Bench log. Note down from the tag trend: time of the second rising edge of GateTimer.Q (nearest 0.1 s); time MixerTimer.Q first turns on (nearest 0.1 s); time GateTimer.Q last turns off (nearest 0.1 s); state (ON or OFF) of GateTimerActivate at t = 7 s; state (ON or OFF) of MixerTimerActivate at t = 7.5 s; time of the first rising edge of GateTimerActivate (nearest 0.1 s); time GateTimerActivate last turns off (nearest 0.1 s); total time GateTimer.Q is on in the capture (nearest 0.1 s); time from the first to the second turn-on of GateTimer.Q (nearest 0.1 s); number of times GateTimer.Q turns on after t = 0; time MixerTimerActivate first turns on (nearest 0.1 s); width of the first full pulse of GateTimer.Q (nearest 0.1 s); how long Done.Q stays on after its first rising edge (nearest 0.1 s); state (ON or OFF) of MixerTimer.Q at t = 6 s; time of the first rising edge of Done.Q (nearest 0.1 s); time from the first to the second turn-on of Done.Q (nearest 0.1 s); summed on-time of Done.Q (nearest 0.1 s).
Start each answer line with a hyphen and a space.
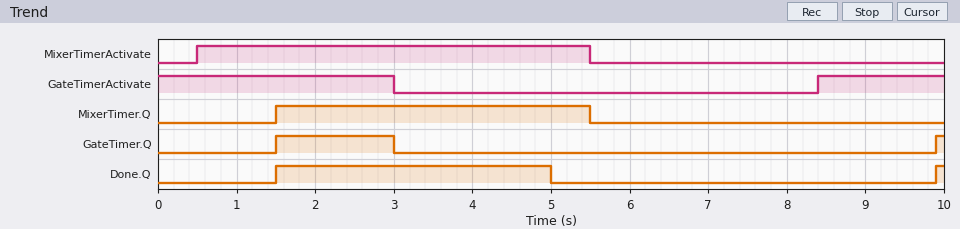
- 9.9 s
- 1.5 s
- 3.0 s
- OFF
- OFF
- 8.4 s
- 3.0 s
- 1.6 s
- 8.4 s
- 2
- 0.5 s
- 1.5 s
- 3.5 s
- OFF
- 1.5 s
- 8.4 s
- 3.6 s
